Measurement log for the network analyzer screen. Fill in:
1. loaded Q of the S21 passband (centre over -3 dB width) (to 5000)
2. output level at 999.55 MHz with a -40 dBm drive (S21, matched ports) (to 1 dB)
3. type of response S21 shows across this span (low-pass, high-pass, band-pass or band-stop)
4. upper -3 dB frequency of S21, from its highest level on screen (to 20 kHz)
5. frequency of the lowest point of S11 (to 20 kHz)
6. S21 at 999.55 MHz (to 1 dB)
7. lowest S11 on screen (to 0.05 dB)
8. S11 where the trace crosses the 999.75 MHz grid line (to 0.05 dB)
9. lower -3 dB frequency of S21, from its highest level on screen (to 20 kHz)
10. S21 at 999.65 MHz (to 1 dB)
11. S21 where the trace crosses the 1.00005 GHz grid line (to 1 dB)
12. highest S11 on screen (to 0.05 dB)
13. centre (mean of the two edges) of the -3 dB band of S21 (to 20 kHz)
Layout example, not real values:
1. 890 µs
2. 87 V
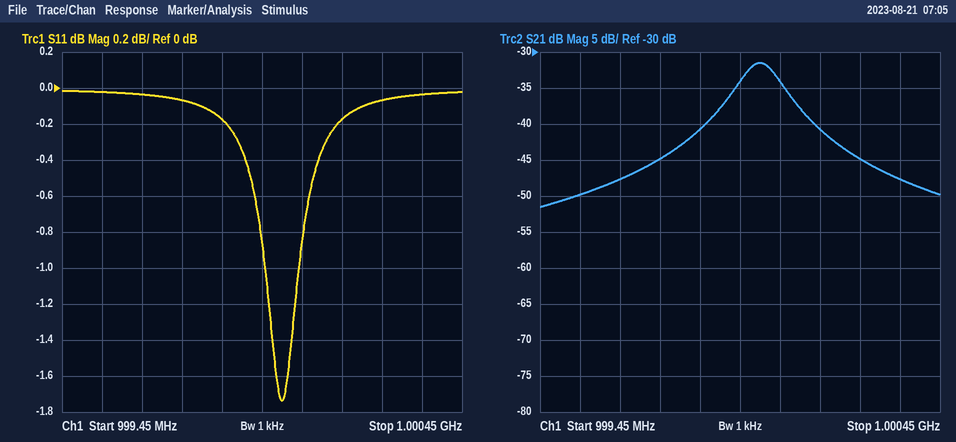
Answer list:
1. 10000
2. -90 dBm
3. band-pass
4. 1.00006 GHz
5. 1.00000 GHz
6. -50 dB
7. -1.75 dB
8. -0.05 dB
9. 999.94 MHz
10. -48 dB
11. -34 dB
12. 0.00 dB
13. 1.00000 GHz
